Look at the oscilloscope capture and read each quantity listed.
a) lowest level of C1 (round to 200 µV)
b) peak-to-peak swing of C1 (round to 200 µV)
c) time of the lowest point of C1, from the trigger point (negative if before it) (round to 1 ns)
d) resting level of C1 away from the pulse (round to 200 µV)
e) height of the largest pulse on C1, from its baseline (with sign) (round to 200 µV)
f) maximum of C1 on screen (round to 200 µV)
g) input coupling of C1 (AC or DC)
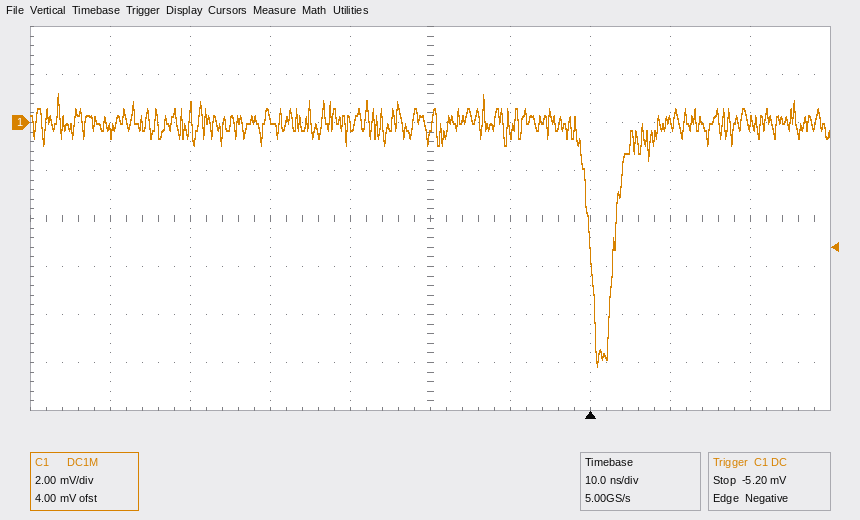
-10.2 mV
11.4 mV
+1 ns
0.0 mV
-10.2 mV
1.2 mV
DC
